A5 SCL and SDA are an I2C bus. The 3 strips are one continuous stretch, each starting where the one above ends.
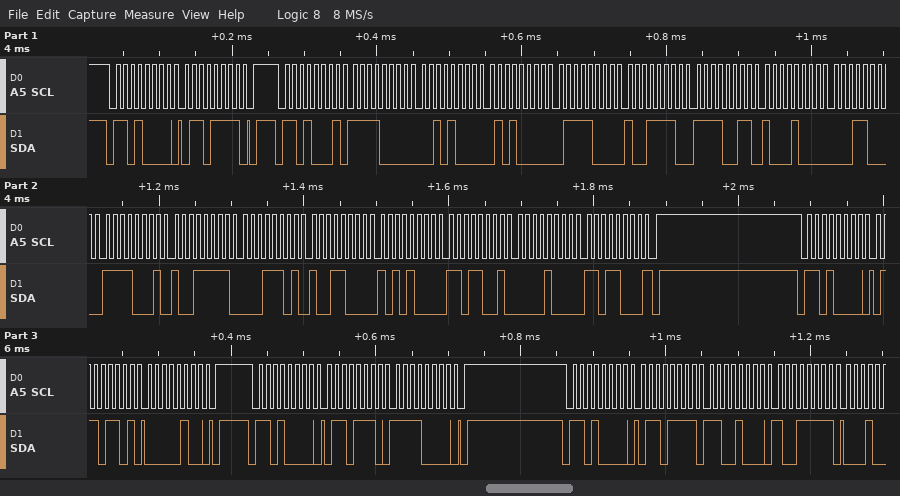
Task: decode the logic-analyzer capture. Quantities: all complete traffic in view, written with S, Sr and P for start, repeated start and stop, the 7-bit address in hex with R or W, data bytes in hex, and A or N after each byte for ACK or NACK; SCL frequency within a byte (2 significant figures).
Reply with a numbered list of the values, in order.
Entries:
1. S 68W A 6F A P S 68R A F0 A 28 A 50 A 78 A 9E A F3 A 88 A 18 A F1 A 9F A 1D A 98 A A8 A D9 A 08 A D8 N P S 68W A 6D A 04 A P S 68W A 6E A F0 A P S 68W A 6F A C8 A 9F A
2. 100 kHz
